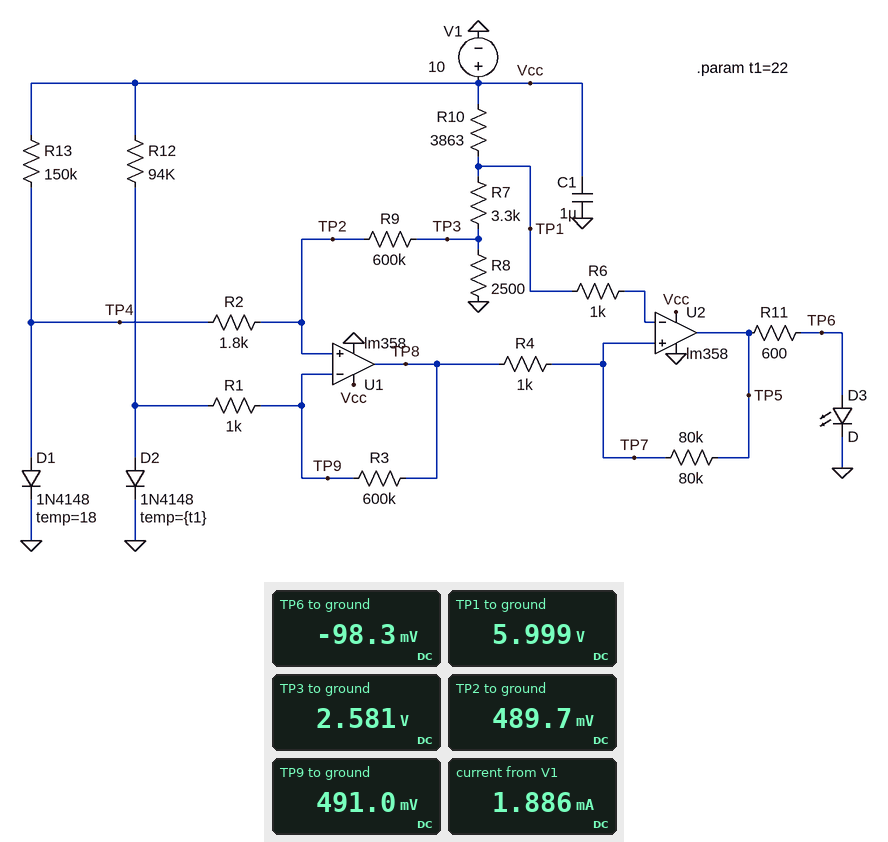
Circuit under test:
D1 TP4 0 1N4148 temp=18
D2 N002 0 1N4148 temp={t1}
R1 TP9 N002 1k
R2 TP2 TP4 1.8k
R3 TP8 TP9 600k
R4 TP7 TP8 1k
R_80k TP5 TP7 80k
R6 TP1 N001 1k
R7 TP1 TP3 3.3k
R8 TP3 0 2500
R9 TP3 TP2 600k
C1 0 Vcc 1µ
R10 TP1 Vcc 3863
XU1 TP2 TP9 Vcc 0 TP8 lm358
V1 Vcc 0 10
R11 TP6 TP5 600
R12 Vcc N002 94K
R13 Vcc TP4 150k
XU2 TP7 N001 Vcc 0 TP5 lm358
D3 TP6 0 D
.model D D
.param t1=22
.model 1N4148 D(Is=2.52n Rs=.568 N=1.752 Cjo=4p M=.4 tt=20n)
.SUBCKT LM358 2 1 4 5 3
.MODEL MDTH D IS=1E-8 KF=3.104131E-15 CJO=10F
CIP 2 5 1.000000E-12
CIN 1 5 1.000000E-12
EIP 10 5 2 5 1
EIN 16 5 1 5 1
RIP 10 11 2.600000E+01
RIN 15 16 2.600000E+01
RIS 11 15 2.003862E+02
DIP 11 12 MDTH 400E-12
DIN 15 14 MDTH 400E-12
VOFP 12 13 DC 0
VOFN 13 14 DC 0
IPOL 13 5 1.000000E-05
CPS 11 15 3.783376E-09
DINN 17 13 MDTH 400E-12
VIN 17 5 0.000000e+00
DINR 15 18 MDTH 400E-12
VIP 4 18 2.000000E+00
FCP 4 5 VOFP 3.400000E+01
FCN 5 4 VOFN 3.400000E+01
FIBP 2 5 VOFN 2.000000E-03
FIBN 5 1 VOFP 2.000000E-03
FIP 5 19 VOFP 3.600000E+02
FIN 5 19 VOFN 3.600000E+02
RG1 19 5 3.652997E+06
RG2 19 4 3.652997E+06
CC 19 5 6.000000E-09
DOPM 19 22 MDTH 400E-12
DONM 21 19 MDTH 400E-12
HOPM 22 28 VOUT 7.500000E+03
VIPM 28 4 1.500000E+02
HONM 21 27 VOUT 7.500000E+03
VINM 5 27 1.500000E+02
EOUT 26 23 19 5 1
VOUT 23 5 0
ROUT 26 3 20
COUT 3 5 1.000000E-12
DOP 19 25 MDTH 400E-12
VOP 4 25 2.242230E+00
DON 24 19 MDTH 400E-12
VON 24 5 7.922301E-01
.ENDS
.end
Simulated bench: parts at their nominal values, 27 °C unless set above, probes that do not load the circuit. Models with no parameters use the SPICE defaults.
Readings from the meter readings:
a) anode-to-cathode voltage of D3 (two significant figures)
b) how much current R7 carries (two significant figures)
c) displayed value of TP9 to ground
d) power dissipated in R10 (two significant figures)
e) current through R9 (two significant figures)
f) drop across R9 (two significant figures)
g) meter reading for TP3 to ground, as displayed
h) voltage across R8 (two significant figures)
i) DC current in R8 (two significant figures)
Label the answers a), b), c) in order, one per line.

a) -98 mV
b) 1.0 mA
c) 491.0 mV
d) 4.1 mW
e) 3.5 µA
f) 2.1 V
g) 2.581 V
h) 2.6 V
i) 1.0 mA
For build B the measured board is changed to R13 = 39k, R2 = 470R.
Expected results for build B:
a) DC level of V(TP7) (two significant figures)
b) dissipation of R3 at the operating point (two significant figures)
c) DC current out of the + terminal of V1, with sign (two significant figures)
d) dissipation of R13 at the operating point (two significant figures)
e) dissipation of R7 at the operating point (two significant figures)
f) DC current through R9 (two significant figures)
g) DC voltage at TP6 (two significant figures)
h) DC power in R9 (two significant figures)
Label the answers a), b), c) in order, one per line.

a) 8.6 V
b) 110 µW
c) -3.1 mA
d) 2.3 mW
e) 3.5 mW
f) 3.4 µA
g) 720 mV
h) 6.9 µW
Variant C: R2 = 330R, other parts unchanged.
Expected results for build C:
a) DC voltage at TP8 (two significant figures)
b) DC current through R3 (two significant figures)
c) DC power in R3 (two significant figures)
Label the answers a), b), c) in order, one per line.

a) -38 mV
b) 880 nA
c) 470 nW
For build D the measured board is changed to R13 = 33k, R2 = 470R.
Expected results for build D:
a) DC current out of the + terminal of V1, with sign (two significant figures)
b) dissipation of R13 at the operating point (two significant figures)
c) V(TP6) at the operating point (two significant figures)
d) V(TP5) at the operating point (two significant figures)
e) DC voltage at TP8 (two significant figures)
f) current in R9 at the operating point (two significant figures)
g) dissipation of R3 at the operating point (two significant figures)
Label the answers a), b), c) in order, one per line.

a) -3.4 mA
b) 2.7 mW
c) 720 mV
d) 8.4 V
e) 8.6 V
f) 3.4 µA
g) 110 µW
